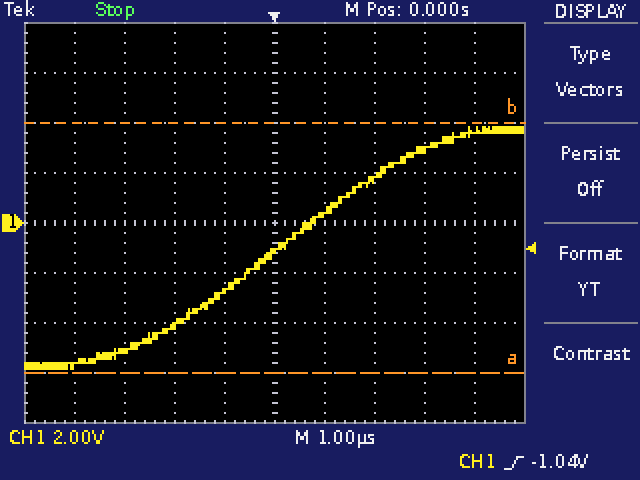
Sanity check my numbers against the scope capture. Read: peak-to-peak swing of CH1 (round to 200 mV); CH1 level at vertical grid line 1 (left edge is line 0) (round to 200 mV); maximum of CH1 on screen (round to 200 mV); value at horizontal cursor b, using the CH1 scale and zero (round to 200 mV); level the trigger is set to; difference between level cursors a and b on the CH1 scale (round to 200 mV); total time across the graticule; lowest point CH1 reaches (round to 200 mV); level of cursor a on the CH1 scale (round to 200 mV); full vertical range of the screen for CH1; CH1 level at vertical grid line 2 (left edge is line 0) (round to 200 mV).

9.6 V
-5.8 V
3.8 V
4.0 V
-1.04 V
10.0 V
10 µs
-5.8 V
-6.0 V
16 V
-5.2 V
